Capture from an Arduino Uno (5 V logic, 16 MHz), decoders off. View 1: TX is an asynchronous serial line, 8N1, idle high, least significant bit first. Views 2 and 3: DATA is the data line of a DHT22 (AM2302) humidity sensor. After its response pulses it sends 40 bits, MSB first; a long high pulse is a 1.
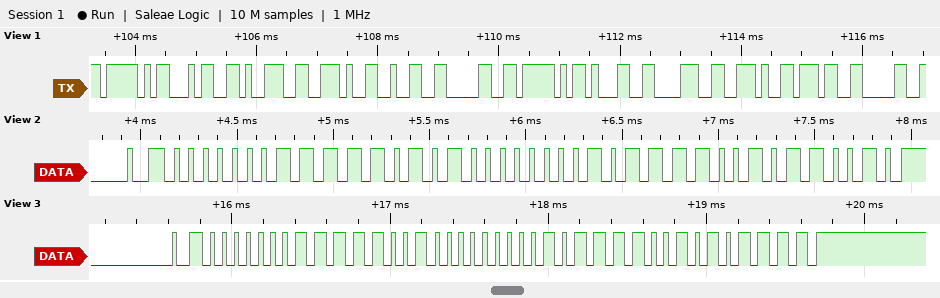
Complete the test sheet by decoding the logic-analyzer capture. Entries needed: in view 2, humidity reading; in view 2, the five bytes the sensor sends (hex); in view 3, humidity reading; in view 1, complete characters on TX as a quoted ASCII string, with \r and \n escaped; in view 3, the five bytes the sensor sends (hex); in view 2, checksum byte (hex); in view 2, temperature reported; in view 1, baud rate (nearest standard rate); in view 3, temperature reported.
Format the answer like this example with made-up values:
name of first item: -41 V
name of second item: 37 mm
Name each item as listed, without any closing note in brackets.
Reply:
in view 2, humidity reading: 50.1 %
in view 2, the five bytes the sensor sends: 01 F5 00 BC B2
in view 3, humidity reading: 49.8 %
in view 1, complete characters on TX as a quoted ASCII string, with \r and \n escaped: "_49.20_18.70"
in view 3, the five bytes the sensor sends: 01 F2 00 BC AF
in view 2, checksum byte: 0xB2
in view 2, temperature reported: 18.8 °C
in view 1, baud rate: 9600 baud
in view 3, temperature reported: 18.8 °C
